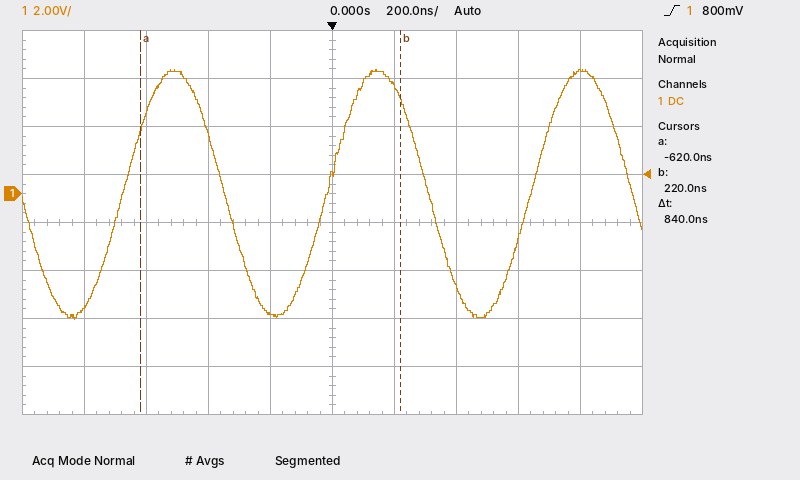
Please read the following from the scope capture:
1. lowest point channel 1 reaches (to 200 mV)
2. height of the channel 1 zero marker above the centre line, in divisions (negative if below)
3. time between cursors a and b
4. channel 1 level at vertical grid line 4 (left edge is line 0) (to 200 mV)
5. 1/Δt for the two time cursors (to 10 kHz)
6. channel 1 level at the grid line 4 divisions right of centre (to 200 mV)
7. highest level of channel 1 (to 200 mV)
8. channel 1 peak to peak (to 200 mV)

-5.2 V
+0.6 div
840 ns
-5.0 V
1.19 MHz
5.2 V
5.2 V
10.4 V
